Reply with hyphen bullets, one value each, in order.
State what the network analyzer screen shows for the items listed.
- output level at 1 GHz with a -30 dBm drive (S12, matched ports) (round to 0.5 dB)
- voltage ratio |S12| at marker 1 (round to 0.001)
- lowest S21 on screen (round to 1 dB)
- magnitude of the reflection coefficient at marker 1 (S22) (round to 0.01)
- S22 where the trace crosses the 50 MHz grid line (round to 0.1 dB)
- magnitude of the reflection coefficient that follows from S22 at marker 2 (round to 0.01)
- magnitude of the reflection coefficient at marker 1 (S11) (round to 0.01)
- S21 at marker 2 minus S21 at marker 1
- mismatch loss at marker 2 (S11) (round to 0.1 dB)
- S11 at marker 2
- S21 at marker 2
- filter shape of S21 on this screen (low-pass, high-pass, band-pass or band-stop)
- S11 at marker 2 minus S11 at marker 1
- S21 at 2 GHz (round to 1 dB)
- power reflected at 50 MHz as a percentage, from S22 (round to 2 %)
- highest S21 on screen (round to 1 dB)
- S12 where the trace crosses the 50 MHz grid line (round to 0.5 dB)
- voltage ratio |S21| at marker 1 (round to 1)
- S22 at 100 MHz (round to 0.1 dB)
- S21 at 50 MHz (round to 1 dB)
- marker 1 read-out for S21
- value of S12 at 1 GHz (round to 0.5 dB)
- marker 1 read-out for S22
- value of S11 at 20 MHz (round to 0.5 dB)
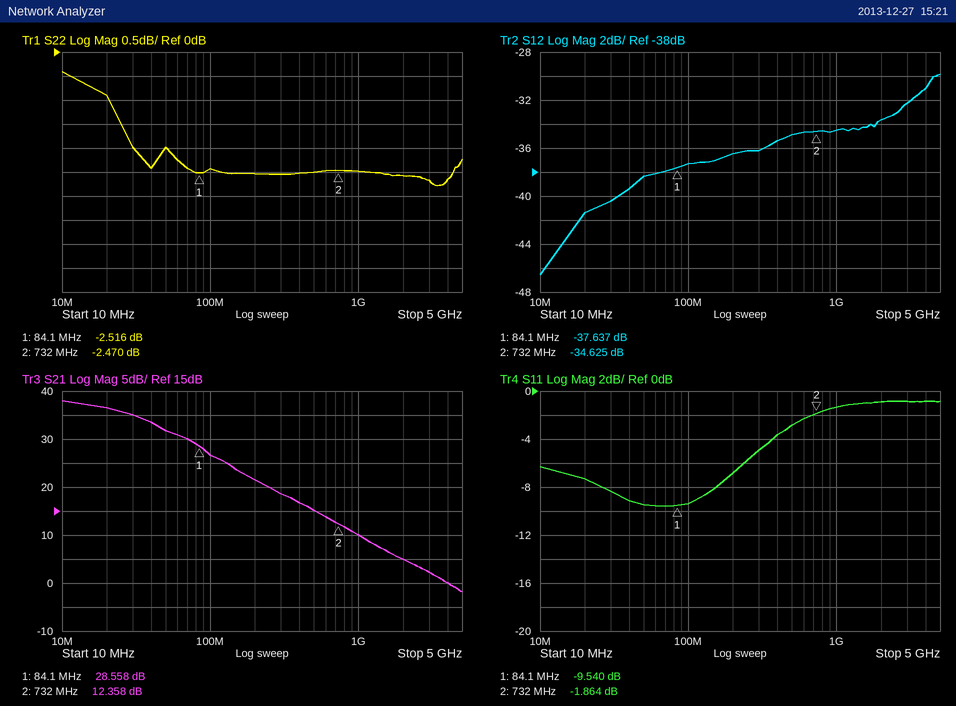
- -64.5 dBm
- 0.013
- -2 dB
- 0.75
- -2.0 dB
- 0.75
- 0.33
- -16.200 dB
- 4.6 dB
- -1.864 dB
- 12.358 dB
- low-pass
- 7.676 dB
- 5 dB
- 64 %
- 38 dB
- -38.5 dB
- 27
- -2.4 dB
- 32 dB
- 28.558 dB
- -34.5 dB
- -2.516 dB
- -7.5 dB
